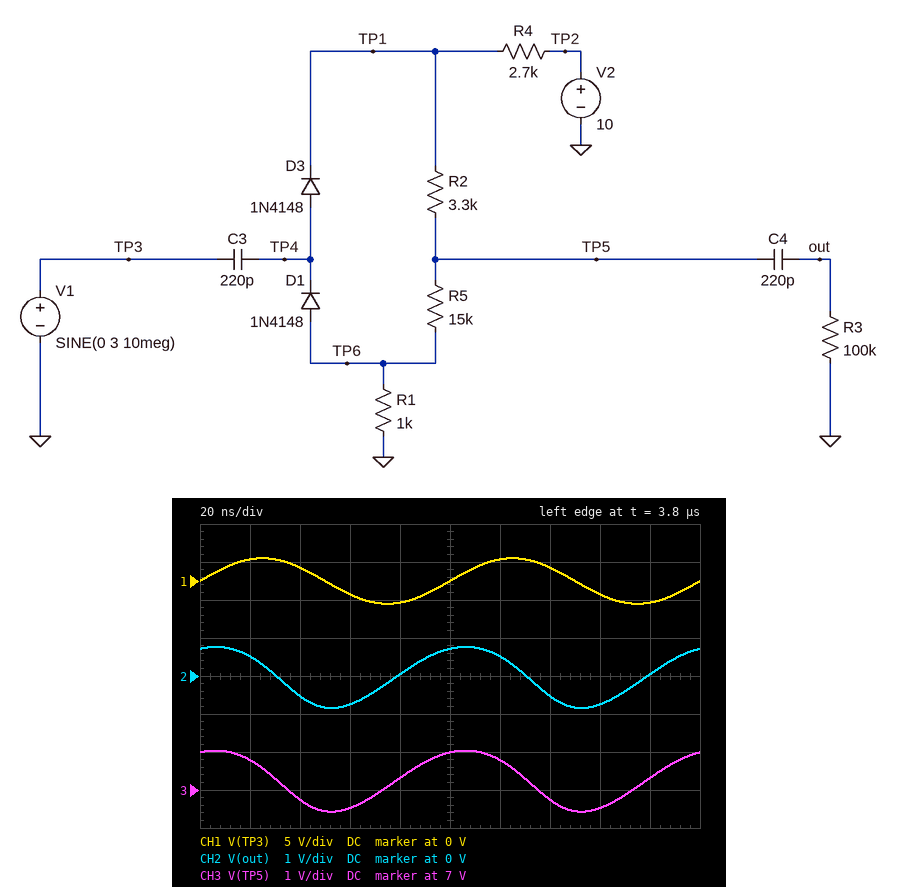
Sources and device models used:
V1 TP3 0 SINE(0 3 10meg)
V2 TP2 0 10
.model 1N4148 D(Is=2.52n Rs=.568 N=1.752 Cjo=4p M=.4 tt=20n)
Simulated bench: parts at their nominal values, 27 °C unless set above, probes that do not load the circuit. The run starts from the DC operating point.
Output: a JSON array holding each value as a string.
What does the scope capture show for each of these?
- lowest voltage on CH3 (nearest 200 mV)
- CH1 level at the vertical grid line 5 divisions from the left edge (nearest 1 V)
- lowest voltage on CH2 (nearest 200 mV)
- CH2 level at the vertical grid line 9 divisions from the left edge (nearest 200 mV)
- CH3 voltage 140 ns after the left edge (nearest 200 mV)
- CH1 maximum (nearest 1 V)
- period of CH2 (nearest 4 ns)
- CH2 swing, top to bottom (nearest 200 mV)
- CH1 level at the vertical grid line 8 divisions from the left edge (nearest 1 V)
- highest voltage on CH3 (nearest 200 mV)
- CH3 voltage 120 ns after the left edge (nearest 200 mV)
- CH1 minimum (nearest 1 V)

["6.4 V", "0 V", "-800 mV", "0 V", "6.8 V", "3 V", "100 ns", "1.6 V", "-2 V", "8.0 V", "7.8 V", "-3 V"]
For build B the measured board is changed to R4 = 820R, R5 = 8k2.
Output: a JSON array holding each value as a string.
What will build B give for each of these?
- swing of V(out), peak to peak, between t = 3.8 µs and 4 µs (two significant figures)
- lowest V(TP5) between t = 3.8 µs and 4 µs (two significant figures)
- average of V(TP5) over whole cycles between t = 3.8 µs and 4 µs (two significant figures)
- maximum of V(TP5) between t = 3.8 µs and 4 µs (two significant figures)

["650 mV", "6.6 V", "6.9 V", "7.2 V"]
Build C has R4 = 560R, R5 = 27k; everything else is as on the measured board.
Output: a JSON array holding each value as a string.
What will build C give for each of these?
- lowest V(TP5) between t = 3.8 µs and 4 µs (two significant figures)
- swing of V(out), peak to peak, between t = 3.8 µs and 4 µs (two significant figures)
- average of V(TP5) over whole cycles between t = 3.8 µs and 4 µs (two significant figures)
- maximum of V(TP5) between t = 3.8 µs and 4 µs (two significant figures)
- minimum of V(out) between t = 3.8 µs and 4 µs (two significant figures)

["8.6 V", "440 mV", "8.8 V", "9.0 V", "-220 mV"]
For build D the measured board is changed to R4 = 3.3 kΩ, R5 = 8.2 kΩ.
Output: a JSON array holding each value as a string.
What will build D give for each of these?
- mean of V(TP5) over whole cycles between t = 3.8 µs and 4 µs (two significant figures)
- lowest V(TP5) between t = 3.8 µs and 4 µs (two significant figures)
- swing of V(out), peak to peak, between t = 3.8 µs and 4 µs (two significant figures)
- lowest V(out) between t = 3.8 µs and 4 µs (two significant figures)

["5.8 V", "4.9 V", "1.7 V", "-920 mV"]
